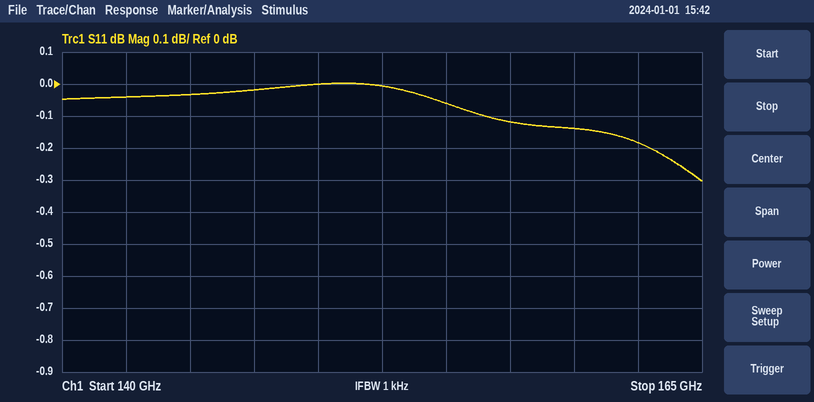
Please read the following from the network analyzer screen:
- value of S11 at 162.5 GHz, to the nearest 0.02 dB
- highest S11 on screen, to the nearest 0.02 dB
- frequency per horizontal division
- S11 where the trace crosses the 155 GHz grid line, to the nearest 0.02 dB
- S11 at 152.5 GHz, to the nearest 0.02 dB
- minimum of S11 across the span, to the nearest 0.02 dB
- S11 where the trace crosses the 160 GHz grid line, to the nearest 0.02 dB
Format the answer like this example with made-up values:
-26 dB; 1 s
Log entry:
-0.18 dB; 0.00 dB; 2.5 GHz; -0.06 dB; 0.00 dB; -0.30 dB; -0.14 dB
